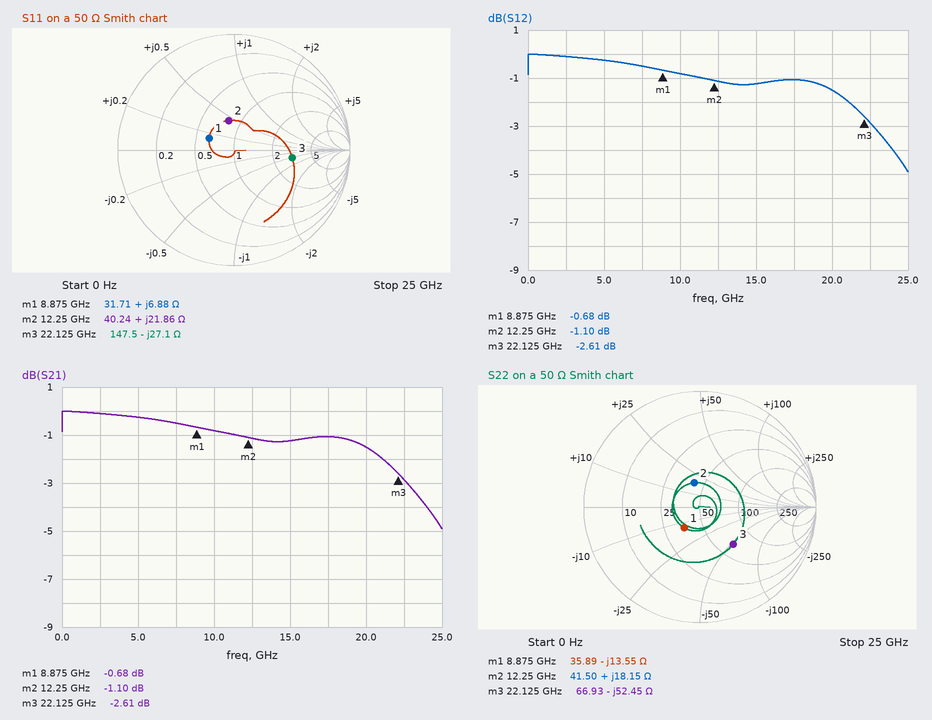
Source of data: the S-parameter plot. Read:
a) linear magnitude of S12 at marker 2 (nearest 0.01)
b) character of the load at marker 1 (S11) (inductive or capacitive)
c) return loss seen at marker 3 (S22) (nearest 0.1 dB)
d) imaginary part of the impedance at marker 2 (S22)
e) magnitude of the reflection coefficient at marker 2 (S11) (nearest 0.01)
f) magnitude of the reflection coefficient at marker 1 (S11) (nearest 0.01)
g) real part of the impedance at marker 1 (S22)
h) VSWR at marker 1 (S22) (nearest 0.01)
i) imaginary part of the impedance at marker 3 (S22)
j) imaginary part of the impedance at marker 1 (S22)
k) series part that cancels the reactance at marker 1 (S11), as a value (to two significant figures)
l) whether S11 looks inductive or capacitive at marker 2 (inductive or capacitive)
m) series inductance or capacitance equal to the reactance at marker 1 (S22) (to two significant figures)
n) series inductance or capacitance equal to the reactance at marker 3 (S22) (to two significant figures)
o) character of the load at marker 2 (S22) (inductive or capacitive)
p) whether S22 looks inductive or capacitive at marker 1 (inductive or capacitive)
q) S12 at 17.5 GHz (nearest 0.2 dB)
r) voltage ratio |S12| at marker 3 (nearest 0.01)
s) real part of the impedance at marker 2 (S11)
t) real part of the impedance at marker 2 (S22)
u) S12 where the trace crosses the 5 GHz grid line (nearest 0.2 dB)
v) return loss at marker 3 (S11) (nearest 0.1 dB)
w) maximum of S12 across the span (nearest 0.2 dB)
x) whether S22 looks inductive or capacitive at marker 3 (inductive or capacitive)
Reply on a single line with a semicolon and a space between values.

0.88; inductive; 7.3 dB; +18.15 Ω; 0.26; 0.24; 35.89 Ω; 1.58; -52.45 Ω; -13.55 Ω; 2.6 pF; inductive; 1.3 pF; 140 fF; inductive; capacitive; -1.0 dB; 0.74; 40.24 Ω; 41.50 Ω; -0.2 dB; 5.9 dB; 0.0 dB; capacitive
